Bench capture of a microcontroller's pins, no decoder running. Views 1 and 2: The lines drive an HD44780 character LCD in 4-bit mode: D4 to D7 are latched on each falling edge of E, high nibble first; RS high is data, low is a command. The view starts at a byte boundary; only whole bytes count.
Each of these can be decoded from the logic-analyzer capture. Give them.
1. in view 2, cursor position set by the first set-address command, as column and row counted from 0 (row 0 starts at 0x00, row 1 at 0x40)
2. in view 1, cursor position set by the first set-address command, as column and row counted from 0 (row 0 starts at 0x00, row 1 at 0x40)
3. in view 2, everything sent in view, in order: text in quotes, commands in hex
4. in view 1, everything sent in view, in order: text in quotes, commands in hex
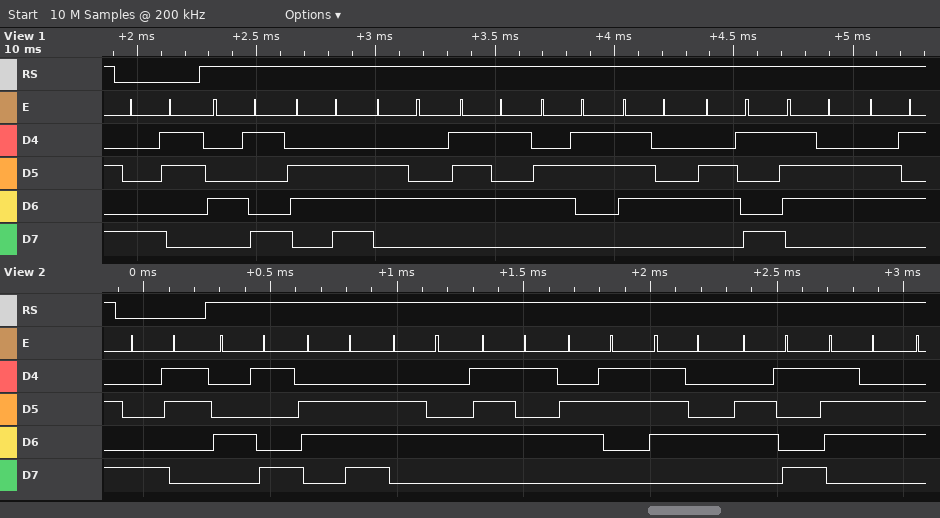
column 3, row 0
column 3, row 0
0x83 "Inductiv"
0x83 "Inductive"
